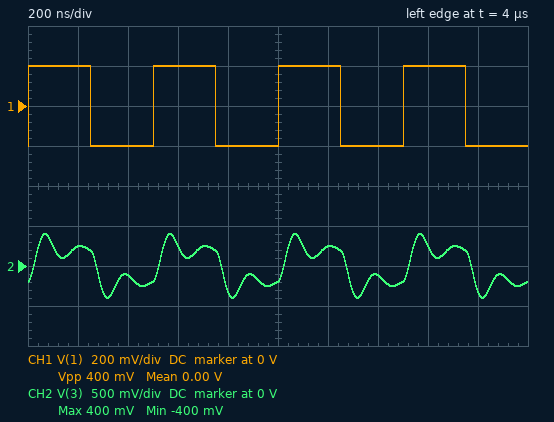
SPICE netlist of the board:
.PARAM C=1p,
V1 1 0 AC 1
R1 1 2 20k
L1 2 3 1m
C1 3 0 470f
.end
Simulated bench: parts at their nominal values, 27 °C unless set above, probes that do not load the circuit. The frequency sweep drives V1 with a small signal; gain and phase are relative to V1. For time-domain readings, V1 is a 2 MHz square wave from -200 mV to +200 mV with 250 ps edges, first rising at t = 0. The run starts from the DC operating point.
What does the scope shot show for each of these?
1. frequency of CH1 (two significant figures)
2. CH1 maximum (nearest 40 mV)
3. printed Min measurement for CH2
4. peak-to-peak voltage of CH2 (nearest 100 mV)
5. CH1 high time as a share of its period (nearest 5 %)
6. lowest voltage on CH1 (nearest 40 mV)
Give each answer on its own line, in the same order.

2.0 MHz
200 mV
-400 mV
800 mV
50 %
-200 mV
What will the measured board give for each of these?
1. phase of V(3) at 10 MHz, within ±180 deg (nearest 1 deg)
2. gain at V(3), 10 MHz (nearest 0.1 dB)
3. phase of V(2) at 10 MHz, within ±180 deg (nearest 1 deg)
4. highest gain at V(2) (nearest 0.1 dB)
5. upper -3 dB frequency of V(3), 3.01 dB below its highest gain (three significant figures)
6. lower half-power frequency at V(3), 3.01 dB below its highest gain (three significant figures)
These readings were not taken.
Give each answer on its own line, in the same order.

-145 deg
-0.3 dB
35 deg
0 dB
8.46 MHz
5.10 MHz
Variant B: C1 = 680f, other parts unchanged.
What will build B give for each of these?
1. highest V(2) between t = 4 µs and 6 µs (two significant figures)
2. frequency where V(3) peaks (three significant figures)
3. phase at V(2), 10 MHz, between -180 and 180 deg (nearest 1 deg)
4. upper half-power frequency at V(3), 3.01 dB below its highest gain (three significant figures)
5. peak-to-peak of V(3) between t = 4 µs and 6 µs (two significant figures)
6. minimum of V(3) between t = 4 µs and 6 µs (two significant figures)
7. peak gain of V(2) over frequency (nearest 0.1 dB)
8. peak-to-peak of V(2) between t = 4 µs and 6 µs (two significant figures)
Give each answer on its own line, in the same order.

270 mV
5.67 MHz
27 deg
7.14 MHz
770 mV
-390 mV
0 dB
540 mV
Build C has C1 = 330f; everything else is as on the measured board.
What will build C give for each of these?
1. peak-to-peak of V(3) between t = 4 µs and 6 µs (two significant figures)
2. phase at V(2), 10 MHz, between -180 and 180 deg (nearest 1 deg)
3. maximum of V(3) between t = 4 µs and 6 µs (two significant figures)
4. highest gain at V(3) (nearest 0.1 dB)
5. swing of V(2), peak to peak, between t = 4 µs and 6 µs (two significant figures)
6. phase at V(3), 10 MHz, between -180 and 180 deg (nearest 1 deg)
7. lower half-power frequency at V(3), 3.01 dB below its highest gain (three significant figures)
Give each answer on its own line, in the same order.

820 mV
54 deg
410 mV
8.9 dB
520 mV
-126 deg
6.65 MHz
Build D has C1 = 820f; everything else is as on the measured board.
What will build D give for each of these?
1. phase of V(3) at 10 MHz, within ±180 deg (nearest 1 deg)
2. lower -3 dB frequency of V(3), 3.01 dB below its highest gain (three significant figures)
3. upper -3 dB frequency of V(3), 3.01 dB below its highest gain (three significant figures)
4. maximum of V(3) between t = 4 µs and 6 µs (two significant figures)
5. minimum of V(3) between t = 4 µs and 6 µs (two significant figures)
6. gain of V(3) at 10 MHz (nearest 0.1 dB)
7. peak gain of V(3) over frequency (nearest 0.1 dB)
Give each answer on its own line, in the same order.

-155 deg
2.98 MHz
6.54 MHz
360 mV
-360 mV
-7.8 dB
5.2 dB
